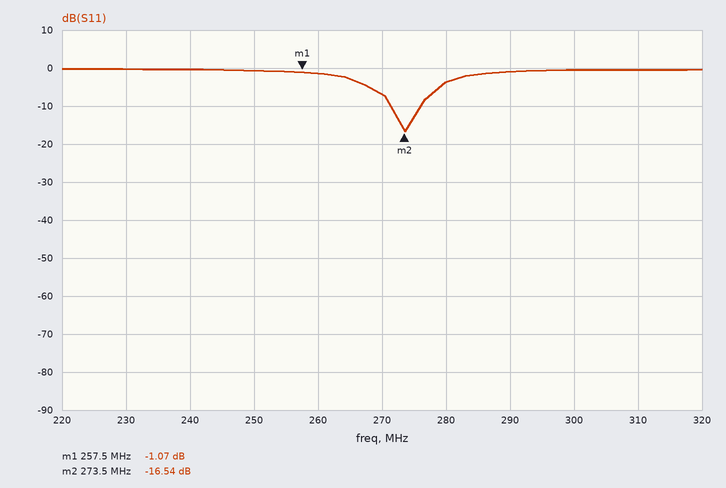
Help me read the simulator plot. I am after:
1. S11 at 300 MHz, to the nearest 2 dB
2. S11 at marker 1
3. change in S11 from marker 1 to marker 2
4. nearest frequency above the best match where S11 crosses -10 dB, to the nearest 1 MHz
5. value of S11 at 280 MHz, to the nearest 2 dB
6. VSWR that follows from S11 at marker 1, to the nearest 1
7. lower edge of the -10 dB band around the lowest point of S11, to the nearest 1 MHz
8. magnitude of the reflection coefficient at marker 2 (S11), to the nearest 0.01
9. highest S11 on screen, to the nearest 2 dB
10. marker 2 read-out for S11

0 dB
-1.07 dB
-15.47 dB
276 MHz
-4 dB
16
271 MHz
0.15
0 dB
-16.54 dB
